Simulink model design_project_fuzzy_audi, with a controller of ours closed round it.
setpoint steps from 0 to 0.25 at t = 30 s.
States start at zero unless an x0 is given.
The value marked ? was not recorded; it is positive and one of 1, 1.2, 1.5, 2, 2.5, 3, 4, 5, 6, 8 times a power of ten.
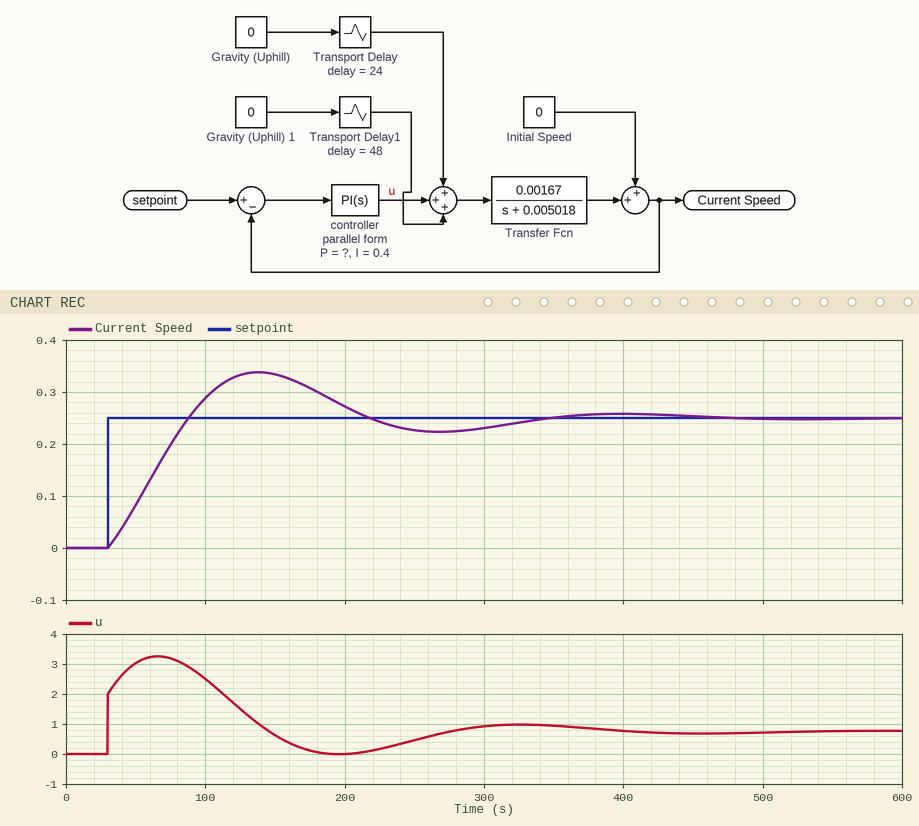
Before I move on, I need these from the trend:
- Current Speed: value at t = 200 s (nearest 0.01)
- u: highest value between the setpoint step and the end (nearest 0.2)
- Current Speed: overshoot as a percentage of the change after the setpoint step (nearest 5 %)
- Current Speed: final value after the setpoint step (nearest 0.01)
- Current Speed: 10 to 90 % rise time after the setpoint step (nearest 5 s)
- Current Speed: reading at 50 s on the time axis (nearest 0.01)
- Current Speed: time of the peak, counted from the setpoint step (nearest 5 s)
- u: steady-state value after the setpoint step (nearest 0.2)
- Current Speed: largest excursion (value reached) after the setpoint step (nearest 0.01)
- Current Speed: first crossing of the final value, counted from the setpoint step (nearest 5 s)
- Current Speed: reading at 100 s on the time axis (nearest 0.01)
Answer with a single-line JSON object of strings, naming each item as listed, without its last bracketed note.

{"Current Speed: value at t = 200 s": "0.27", "u: highest value between the setpoint step and the end": "3.2", "Current Speed: overshoot as a percentage of the change after the setpoint step": "35 %", "Current Speed: final value after the setpoint step": "0.25", "Current Speed: 10 to 90 % rise time after the setpoint step": "45 s", "Current Speed: reading at 50 s on the time axis": "0.08", "Current Speed: time of the peak, counted from the setpoint step": "110 s", "u: steady-state value after the setpoint step": "0.8", "Current Speed: largest excursion (value reached) after the setpoint step": "0.34", "Current Speed: first crossing of the final value, counted from the setpoint step": "60 s", "Current Speed: reading at 100 s on the time axis": "0.29"}
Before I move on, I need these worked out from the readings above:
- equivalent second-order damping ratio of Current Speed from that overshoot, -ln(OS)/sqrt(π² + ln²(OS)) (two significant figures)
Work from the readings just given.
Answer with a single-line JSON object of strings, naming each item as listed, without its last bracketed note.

{"equivalent second-order damping ratio of Current Speed from that overshoot, -ln(OS)/sqrt(π² + ln²(OS))": "0.32"}
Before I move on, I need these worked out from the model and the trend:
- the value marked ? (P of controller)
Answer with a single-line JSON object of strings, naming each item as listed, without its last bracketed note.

{"the value marked ?": "8"}
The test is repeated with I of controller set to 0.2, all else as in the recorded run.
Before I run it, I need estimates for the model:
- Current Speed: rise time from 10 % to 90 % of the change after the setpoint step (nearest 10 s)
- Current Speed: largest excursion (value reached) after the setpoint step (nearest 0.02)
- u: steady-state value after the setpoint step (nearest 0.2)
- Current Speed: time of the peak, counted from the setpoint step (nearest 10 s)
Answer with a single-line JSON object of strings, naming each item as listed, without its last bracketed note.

{"Current Speed: rise time from 10 % to 90 % of the change after the setpoint step": "60 s", "Current Speed: largest excursion (value reached) after the setpoint step": "0.30", "u: steady-state value after the setpoint step": "0.8", "Current Speed: time of the peak, counted from the setpoint step": "150 s"}
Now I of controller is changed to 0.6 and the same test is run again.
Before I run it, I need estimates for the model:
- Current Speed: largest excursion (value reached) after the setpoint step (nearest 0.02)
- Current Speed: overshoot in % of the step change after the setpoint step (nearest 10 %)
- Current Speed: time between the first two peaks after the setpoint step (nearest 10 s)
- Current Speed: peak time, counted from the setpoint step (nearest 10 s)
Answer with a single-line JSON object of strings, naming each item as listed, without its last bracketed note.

{"Current Speed: largest excursion (value reached) after the setpoint step": "0.36", "Current Speed: overshoot in % of the step change after the setpoint step": "40 %", "Current Speed: time between the first two peaks after the setpoint step": "210 s", "Current Speed: peak time, counted from the setpoint step": "90 s"}
